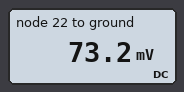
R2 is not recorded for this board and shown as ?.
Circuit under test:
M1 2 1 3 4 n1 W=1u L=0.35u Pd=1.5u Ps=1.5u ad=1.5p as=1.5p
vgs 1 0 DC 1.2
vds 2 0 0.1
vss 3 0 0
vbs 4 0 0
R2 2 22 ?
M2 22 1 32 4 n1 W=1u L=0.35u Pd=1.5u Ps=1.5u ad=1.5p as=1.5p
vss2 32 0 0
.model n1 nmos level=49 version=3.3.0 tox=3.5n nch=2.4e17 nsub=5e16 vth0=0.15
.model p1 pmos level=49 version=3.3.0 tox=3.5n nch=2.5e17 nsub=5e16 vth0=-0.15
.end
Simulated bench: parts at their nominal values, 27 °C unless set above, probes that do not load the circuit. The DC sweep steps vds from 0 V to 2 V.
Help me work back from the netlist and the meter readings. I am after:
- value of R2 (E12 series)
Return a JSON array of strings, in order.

["560 Ω"]
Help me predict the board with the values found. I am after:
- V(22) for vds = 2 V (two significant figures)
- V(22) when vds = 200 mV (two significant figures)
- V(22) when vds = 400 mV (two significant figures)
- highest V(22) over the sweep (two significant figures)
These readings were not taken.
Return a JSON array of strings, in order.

["1.9 V", "150 mV", "320 mV", "1.9 V"]
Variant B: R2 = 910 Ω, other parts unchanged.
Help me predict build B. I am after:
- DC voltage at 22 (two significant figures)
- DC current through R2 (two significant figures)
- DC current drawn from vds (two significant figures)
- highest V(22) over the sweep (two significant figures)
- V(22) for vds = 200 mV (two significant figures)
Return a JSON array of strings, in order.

["62 mV", "41 µA", "100 µA", "1.8 V", "130 mV"]
